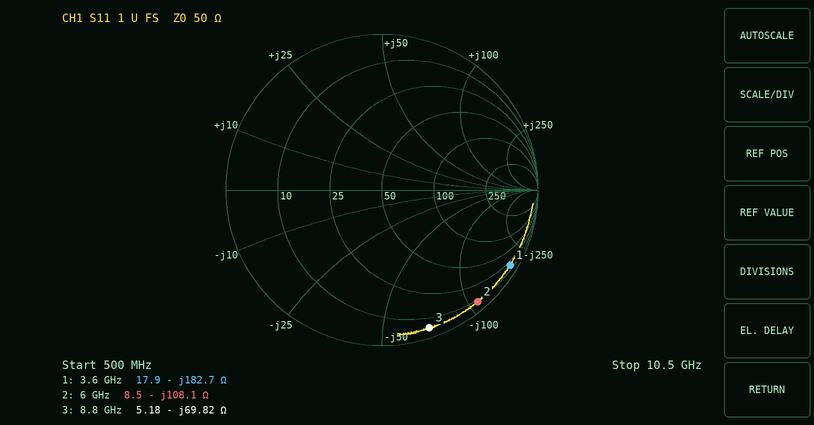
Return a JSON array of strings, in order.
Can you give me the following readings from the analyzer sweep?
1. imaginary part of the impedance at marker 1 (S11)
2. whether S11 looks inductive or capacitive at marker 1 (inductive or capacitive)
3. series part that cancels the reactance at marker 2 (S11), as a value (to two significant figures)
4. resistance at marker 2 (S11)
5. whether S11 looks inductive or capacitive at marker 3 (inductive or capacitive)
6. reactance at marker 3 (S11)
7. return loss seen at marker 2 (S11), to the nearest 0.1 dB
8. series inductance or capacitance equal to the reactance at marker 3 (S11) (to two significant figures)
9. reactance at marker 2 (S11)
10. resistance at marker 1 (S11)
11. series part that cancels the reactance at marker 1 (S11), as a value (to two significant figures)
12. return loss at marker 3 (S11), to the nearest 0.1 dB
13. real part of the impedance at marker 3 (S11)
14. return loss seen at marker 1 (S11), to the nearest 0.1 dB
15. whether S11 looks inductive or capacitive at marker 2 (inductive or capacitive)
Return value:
["-182.7 Ω", "capacitive", "2.9 nH", "8.5 Ω", "capacitive", "-69.82 Ω", "0.5 dB", "260 fF", "-108.1 Ω", "17.9 Ω", "8.1 nH", "0.6 dB", "5.18 Ω", "0.4 dB", "capacitive"]
